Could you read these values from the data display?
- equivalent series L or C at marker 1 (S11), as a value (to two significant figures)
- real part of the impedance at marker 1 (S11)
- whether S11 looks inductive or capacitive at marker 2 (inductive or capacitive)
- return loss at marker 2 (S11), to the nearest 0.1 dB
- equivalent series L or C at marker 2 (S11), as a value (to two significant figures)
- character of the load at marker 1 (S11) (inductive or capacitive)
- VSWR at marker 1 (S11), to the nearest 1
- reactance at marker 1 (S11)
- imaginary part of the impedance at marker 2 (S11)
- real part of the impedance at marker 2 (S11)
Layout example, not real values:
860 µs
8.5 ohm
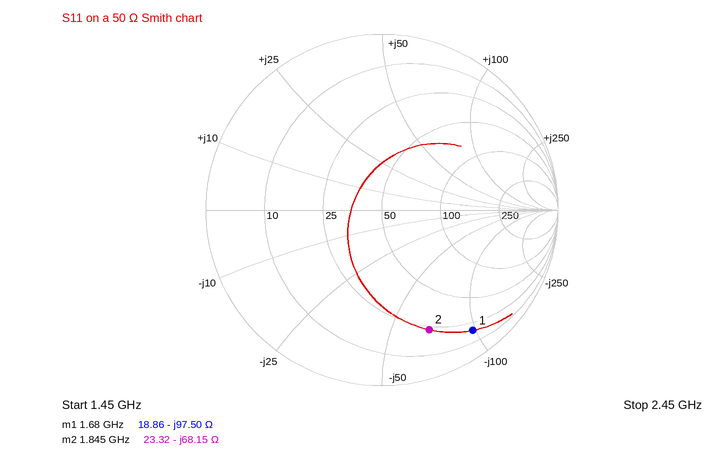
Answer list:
970 fF
18.86 Ω
capacitive
2.7 dB
1.3 pF
capacitive
13
-97.50 Ω
-68.15 Ω
23.32 Ω
